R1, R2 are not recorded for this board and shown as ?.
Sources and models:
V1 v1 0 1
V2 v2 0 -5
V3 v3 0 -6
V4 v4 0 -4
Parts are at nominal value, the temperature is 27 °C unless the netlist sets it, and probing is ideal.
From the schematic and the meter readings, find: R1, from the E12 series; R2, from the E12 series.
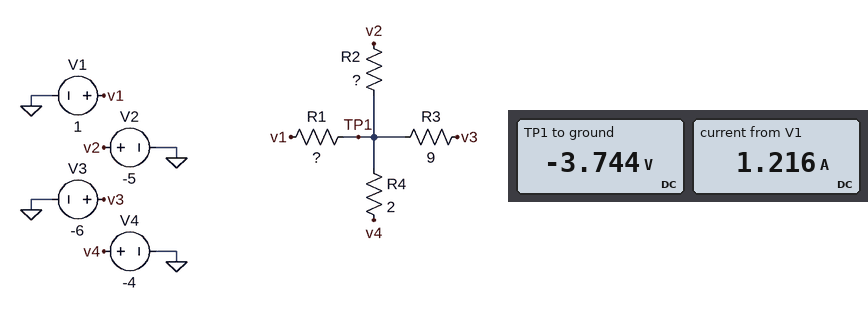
3.9 Ω
1.5 Ω
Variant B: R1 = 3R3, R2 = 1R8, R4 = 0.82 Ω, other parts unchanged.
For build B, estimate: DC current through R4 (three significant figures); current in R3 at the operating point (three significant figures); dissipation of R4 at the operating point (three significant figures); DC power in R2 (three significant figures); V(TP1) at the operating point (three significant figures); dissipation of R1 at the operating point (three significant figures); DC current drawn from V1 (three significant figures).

411 mA
260 mA
138 mW
993 mW
-3.66 V
6.59 W
1.41 A
